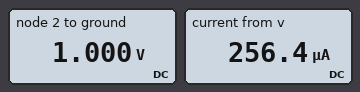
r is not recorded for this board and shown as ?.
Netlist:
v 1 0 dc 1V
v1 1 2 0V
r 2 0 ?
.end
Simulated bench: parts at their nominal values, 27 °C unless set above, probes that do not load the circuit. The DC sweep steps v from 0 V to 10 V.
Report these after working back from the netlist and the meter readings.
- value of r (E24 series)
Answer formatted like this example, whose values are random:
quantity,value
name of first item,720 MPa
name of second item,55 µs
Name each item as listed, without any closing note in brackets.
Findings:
quantity,value
value of r,3.9 kΩ
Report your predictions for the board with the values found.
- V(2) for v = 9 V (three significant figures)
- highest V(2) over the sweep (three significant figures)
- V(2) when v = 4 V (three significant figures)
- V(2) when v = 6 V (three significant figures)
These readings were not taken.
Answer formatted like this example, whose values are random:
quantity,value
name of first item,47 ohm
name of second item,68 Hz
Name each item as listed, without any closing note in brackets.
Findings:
quantity,value
V(2) for v = 9 V,9.00 V
highest V(2) over the sweep,10.0 V
V(2) when v = 4 V,4.00 V
V(2) when v = 6 V,6.00 V
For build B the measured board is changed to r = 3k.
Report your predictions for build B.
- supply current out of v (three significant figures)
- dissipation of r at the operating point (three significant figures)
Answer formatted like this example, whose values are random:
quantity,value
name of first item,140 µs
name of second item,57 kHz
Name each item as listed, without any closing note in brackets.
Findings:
quantity,value
supply current out of v,333 µA
dissipation of r at the operating point,333 µW
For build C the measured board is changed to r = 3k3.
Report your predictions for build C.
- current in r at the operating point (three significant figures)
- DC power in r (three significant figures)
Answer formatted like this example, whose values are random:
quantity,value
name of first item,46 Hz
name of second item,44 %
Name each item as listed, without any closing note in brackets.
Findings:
quantity,value
current in r at the operating point,303 µA
DC power in r,303 µW
